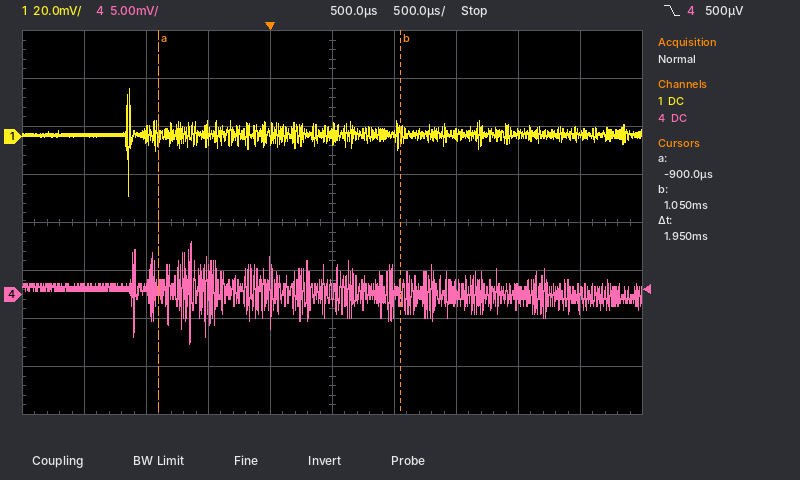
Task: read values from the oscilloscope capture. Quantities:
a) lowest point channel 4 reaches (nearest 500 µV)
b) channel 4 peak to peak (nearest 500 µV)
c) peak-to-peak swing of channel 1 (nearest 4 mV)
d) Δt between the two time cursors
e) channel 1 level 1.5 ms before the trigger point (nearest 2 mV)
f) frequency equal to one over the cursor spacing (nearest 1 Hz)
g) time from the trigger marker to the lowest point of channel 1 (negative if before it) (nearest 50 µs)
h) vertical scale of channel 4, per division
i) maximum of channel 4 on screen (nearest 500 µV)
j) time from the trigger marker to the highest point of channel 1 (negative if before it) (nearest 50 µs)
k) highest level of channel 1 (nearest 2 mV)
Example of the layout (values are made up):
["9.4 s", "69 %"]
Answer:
["-5.0 mV", "10.5 mV", "44 mV", "1.95 ms", "0 mV", "513 Hz", "-1.15 ms", "5 mV", "5.5 mV", "-1.15 ms", "20 mV"]
